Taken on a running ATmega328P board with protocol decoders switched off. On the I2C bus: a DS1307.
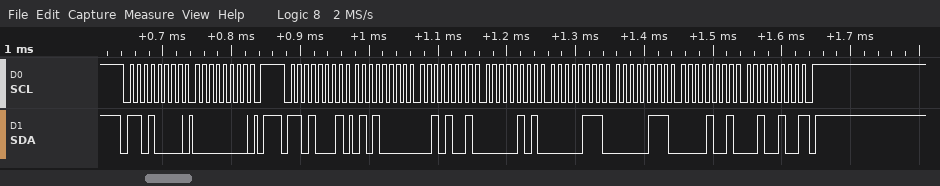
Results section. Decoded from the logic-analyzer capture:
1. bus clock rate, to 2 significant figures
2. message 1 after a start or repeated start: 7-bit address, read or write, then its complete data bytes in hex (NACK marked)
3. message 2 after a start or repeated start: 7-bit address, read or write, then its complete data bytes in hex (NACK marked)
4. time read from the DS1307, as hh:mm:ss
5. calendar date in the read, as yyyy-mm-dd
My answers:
100 kHz
0x68 write: 00
0x68 read: 50 29 05 07 07 09 24 NACK
05:29:50
2024-09-07
